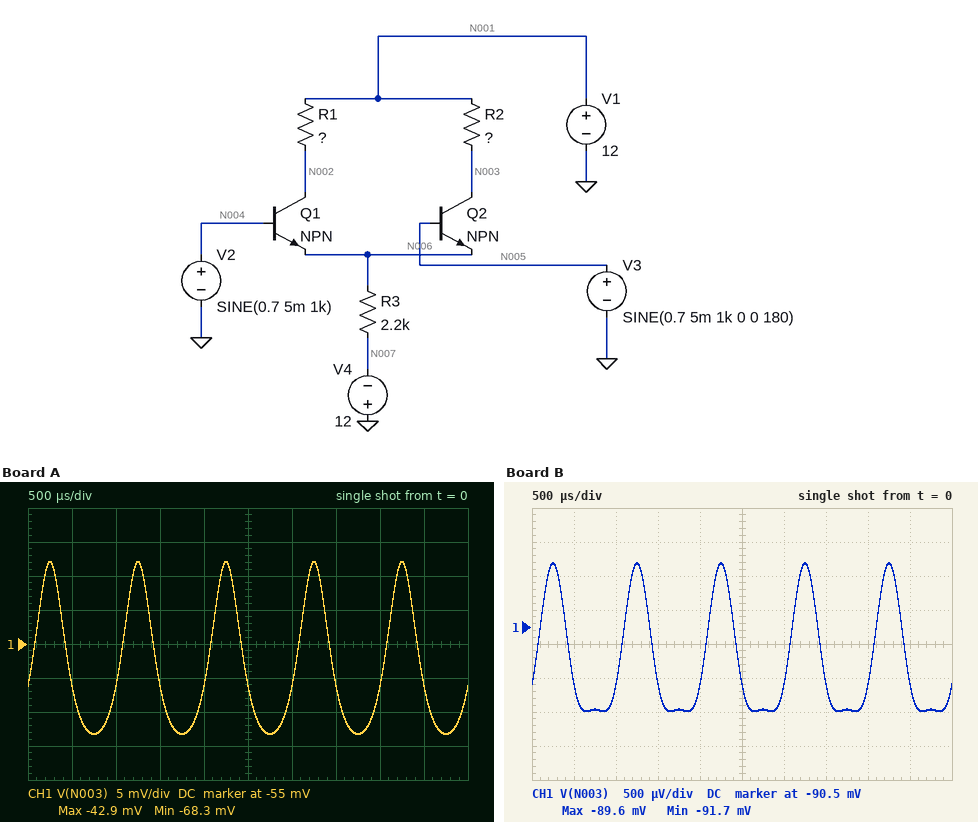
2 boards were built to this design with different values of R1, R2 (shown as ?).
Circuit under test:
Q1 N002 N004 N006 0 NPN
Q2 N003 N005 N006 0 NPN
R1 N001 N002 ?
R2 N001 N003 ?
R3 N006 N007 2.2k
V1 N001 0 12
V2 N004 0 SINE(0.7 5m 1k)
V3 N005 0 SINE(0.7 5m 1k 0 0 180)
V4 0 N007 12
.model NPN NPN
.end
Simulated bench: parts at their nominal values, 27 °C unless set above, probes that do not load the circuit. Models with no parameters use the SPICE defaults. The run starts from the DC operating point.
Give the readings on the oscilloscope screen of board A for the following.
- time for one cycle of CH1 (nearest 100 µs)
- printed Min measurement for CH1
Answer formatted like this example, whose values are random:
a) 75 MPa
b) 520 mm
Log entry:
a) 1.0 ms
b) -68.3 mV
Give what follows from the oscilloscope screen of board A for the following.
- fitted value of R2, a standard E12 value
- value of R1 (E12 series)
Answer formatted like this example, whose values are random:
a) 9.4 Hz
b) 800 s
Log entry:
a) 4.7 kΩ
b) 22 kΩ
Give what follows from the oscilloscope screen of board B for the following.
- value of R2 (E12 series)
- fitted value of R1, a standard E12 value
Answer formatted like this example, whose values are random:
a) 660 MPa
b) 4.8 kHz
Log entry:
a) 15 kΩ
b) 27 kΩ
